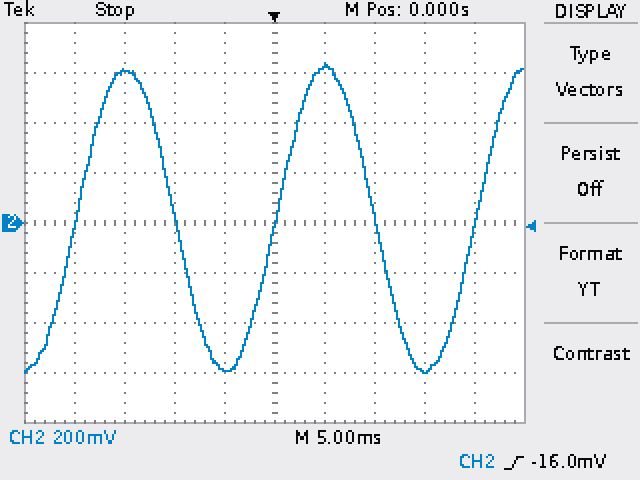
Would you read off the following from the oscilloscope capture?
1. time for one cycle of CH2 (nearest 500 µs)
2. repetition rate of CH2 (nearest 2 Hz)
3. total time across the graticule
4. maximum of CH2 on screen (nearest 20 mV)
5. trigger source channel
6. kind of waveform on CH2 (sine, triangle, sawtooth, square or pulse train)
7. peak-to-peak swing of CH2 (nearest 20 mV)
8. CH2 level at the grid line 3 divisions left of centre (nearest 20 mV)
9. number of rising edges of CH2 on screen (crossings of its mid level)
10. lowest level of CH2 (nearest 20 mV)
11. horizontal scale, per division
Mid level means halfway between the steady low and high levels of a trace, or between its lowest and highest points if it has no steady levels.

20.0 ms
50 Hz
50 ms
640 mV
CH2
sine
1.24 V
600 mV
3
-600 mV
5 ms
